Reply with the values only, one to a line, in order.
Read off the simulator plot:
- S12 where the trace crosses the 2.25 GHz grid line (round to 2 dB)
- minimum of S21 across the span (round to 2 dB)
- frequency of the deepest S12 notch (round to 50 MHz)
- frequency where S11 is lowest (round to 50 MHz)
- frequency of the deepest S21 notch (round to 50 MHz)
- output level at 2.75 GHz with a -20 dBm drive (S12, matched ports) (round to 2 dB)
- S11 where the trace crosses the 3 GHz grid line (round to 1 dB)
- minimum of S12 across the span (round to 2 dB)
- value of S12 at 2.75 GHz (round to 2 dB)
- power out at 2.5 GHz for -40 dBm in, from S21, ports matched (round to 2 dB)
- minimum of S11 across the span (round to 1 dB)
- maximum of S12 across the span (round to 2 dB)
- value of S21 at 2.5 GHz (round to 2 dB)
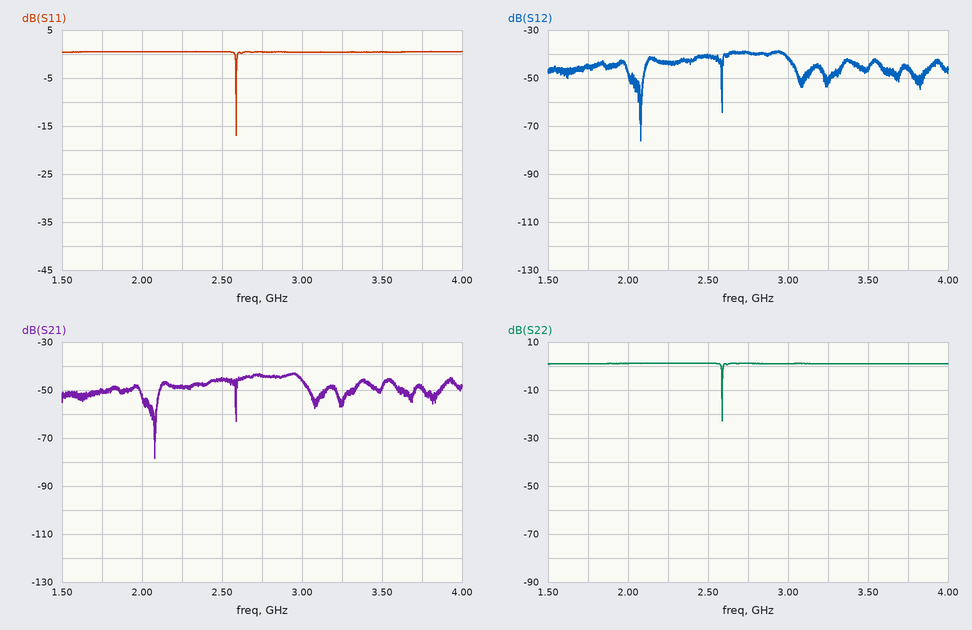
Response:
-44 dB
-78 dB
2.10 GHz
2.60 GHz
2.10 GHz
-60 dBm
0 dB
-76 dB
-40 dB
-86 dBm
-17 dB
-38 dB
-46 dB
